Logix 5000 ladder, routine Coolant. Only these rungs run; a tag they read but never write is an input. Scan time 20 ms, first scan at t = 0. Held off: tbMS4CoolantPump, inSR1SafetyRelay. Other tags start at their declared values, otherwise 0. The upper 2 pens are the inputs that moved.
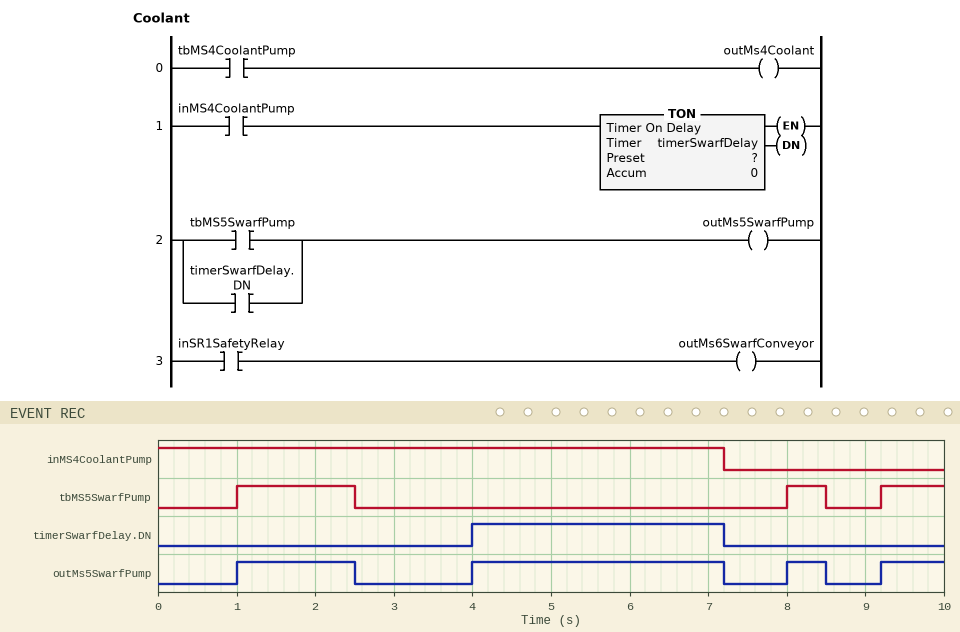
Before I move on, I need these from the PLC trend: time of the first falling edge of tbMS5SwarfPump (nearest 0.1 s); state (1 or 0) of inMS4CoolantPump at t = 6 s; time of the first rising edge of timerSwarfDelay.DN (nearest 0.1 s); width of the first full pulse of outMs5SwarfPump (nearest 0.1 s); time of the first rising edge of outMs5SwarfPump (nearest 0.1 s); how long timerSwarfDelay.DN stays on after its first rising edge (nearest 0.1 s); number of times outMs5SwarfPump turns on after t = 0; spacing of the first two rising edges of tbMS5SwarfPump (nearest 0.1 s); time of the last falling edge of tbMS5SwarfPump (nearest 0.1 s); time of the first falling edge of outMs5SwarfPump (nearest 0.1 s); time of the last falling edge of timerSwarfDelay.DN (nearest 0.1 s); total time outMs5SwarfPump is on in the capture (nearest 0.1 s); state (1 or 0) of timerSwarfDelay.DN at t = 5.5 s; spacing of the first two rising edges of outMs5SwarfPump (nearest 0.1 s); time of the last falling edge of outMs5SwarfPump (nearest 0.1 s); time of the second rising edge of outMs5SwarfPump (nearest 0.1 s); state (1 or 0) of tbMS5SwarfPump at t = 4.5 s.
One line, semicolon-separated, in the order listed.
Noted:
2.5 s; 1; 4.0 s; 1.5 s; 1.0 s; 3.2 s; 4; 7.0 s; 8.5 s; 2.5 s; 7.2 s; 6.0 s; 1; 3.0 s; 8.5 s; 4.0 s; 0
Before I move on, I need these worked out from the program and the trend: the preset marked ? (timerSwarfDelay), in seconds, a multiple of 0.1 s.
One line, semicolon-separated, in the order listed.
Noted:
4.0 s
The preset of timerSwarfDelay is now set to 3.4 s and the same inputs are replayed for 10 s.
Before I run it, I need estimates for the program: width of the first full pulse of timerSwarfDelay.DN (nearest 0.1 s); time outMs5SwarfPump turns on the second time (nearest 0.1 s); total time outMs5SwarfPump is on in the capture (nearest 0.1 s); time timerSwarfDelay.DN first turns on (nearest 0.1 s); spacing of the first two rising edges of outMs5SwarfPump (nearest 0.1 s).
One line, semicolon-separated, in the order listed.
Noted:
3.8 s; 3.4 s; 6.6 s; 3.4 s; 2.4 s
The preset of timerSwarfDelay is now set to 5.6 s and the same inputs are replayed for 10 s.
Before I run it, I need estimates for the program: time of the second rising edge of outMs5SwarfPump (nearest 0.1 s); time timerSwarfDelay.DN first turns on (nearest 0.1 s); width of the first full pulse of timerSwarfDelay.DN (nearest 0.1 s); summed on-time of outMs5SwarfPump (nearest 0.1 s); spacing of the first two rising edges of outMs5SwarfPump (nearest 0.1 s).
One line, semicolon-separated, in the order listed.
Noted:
5.6 s; 5.6 s; 1.6 s; 4.4 s; 4.6 s
